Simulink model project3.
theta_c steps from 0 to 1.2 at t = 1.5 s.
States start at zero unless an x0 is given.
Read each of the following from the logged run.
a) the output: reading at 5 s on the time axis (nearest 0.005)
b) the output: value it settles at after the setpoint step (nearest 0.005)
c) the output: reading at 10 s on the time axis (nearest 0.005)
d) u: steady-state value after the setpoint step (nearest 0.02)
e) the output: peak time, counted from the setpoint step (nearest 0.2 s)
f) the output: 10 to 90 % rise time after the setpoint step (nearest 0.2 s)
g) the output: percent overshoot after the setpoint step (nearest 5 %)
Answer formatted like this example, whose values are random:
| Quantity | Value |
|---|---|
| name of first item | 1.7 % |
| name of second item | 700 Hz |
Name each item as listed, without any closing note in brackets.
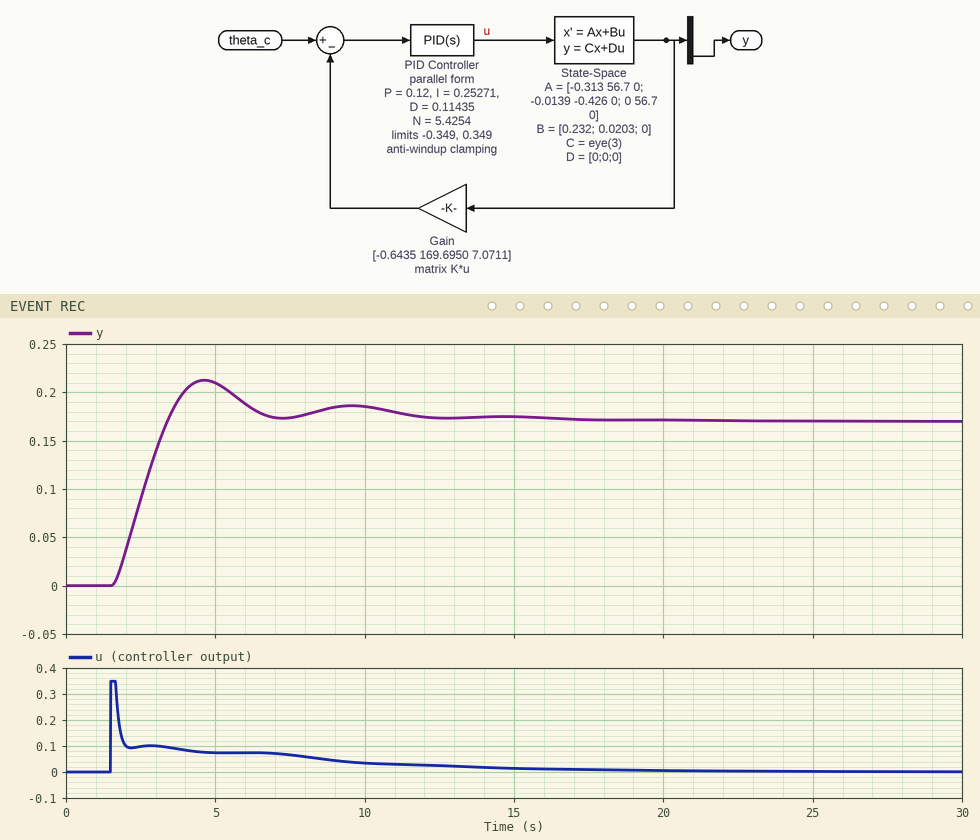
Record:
| Quantity | Value |
|---|---|
| the output: reading at 5 s on the time axis | 0.210 |
| the output: value it settles at after the setpoint step | 0.170 |
| the output: reading at 10 s on the time axis | 0.185 |
| u: steady-state value after the setpoint step | 0.00 |
| the output: peak time, counted from the setpoint step | 3.2 s |
| the output: 10 to 90 % rise time after the setpoint step | 1.4 s |
| the output: percent overshoot after the setpoint step | 25 % |
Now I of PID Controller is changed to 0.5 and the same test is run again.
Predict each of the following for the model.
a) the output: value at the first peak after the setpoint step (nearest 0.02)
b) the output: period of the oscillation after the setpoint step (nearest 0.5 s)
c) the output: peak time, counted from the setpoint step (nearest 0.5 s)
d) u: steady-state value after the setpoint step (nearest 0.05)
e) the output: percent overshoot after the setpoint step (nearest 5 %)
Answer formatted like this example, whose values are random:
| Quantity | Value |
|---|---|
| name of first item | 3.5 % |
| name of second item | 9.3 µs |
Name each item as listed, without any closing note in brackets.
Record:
| Quantity | Value |
|---|---|
| the output: value at the first peak after the setpoint step | 0.24 |
| the output: period of the oscillation after the setpoint step | 4.0 s |
| the output: peak time, counted from the setpoint step | 2.5 s |
| u: steady-state value after the setpoint step | 0.00 |
| the output: percent overshoot after the setpoint step | 40 % |
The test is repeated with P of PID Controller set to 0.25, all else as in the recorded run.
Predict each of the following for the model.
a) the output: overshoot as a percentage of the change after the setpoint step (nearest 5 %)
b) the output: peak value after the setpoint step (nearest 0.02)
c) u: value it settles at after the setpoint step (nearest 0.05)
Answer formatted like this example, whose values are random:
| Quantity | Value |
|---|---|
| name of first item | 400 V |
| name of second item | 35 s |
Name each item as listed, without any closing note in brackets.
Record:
| Quantity | Value |
|---|---|
| the output: overshoot as a percentage of the change after the setpoint step | 15 % |
| the output: peak value after the setpoint step | 0.20 |
| u: value it settles at after the setpoint step | 0.00 |
